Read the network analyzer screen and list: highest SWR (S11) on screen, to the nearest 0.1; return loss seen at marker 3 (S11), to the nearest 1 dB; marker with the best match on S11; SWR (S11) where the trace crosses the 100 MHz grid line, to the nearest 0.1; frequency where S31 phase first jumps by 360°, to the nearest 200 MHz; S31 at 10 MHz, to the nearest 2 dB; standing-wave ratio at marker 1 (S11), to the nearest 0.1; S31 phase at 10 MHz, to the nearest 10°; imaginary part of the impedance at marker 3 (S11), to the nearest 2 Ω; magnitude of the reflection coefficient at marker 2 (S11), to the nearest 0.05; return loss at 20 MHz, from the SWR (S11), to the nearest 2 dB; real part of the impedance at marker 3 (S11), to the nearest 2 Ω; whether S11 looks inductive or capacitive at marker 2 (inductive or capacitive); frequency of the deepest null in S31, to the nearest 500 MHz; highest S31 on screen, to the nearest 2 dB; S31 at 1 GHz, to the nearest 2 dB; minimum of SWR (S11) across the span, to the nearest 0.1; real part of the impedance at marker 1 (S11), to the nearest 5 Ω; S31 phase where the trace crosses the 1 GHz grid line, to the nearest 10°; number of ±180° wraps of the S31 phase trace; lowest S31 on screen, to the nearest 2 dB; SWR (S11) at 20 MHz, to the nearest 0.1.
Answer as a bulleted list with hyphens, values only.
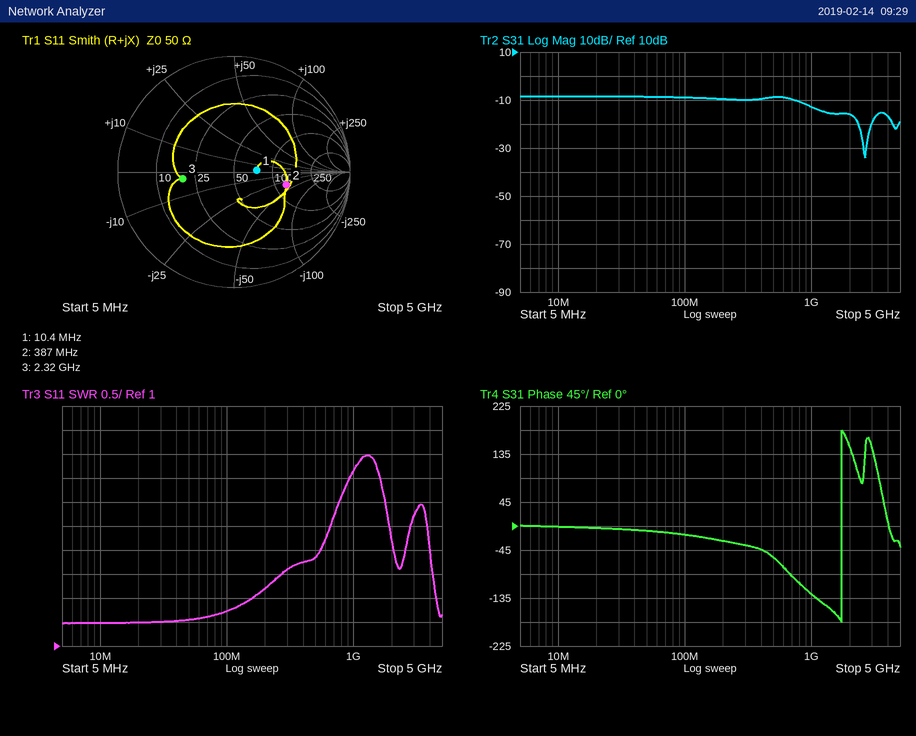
- 5.0
- 7 dB
- marker 1
- 1.7
- 1.8 GHz
- -8 dB
- 1.5
- 0°
- -2 Ω
- 0.45
- 14 dB
- 20 Ω
- capacitive
- 2.5 GHz
- -8 dB
- -12 dB
- 1.5
- 75 Ω
- -130°
- 1
- -34 dB
- 1.5
